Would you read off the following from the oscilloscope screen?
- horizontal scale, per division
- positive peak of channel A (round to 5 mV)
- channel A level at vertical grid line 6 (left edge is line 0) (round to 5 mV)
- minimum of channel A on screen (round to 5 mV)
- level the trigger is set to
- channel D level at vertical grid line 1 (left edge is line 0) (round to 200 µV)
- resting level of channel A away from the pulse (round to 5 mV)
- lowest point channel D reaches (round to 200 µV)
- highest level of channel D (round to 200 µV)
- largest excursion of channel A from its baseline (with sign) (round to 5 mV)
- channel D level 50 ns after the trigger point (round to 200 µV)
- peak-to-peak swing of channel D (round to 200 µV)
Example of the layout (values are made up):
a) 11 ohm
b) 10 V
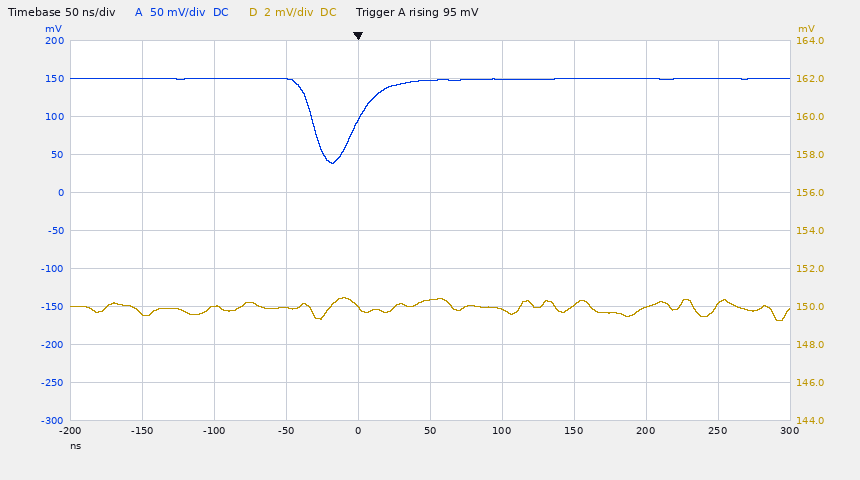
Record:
a) 50 ns
b) 150 mV
c) 150 mV
d) 40 mV
e) 95 mV
f) 149.6 mV
g) 150 mV
h) 149.2 mV
i) 150.4 mV
j) -110 mV
k) 150.4 mV
l) 1.2 mV
